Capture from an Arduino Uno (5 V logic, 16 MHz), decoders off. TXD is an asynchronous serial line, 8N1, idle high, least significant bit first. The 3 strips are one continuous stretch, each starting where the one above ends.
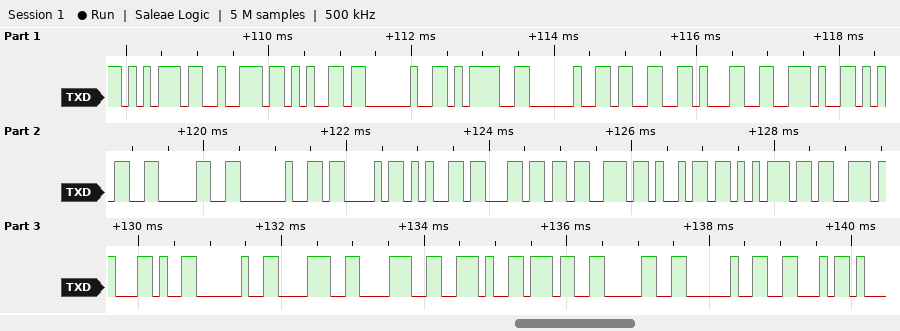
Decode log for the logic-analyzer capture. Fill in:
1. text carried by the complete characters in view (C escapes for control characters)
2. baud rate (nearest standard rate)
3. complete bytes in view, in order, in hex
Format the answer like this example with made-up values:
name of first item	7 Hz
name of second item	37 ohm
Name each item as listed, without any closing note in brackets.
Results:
text carried by the complete characters in view	"ure = 31.50 Celsius, 88.70 F"
baud rate	9600 baud
complete bytes in view, in order, in hex	75 72 65 20 3D 20 33 31 2E 35 30 20 43 65 6C 73 69 75 73 2C 20 38 38 2E 37 30 20 46
